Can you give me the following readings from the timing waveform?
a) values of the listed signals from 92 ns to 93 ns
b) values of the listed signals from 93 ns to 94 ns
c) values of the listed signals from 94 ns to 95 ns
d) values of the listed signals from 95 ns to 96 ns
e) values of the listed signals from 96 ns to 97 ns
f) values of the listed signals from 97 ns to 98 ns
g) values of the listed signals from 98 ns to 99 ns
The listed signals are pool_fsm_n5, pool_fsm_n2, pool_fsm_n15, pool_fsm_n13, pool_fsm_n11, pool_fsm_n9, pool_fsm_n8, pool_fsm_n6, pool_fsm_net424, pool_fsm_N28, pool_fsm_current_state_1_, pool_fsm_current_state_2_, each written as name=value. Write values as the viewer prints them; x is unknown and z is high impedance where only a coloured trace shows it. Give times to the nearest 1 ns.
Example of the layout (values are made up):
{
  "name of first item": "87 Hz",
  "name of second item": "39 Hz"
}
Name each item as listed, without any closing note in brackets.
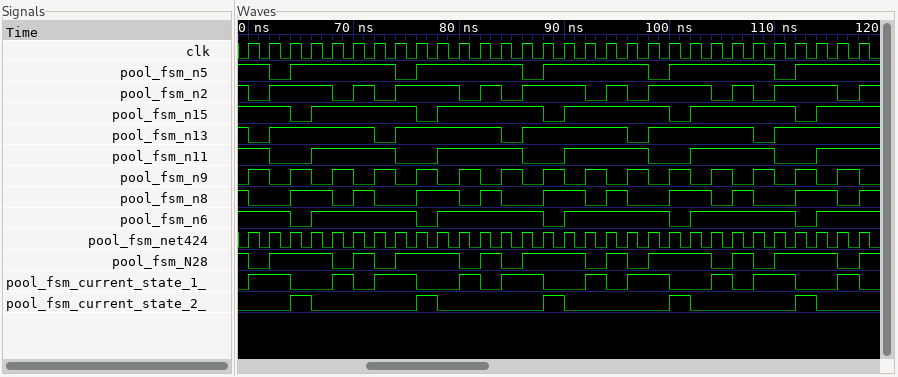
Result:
{
  "values of the listed signals from 92 ns to 93 ns": "pool_fsm_n5=1, pool_fsm_n2=0, pool_fsm_n15=1, pool_fsm_n13=1, pool_fsm_n11=1, pool_fsm_n9=1, pool_fsm_n8=0, pool_fsm_n6=1, pool_fsm_net424=1, pool_fsm_N28=0, pool_fsm_current_state_1_=1, pool_fsm_current_state_2_=0",
  "values of the listed signals from 93 ns to 94 ns": "pool_fsm_n5=1, pool_fsm_n2=0, pool_fsm_n15=1, pool_fsm_n13=1, pool_fsm_n11=1, pool_fsm_n9=1, pool_fsm_n8=0, pool_fsm_n6=1, pool_fsm_net424=0, pool_fsm_N28=0, pool_fsm_current_state_1_=1, pool_fsm_current_state_2_=0",
  "values of the listed signals from 94 ns to 95 ns": "pool_fsm_n5=1, pool_fsm_n2=1, pool_fsm_n15=1, pool_fsm_n13=1, pool_fsm_n11=1, pool_fsm_n9=0, pool_fsm_n8=1, pool_fsm_n6=1, pool_fsm_net424=1, pool_fsm_N28=1, pool_fsm_current_state_1_=0, pool_fsm_current_state_2_=0",
  "values of the listed signals from 95 ns to 96 ns": "pool_fsm_n5=1, pool_fsm_n2=1, pool_fsm_n15=1, pool_fsm_n13=1, pool_fsm_n11=1, pool_fsm_n9=0, pool_fsm_n8=1, pool_fsm_n6=1, pool_fsm_net424=0, pool_fsm_N28=1, pool_fsm_current_state_1_=0, pool_fsm_current_state_2_=0",
  "values of the listed signals from 96 ns to 97 ns": "pool_fsm_n5=1, pool_fsm_n2=0, pool_fsm_n15=1, pool_fsm_n13=0, pool_fsm_n11=1, pool_fsm_n9=1, pool_fsm_n8=0, pool_fsm_n6=1, pool_fsm_net424=1, pool_fsm_N28=0, pool_fsm_current_state_1_=1, pool_fsm_current_state_2_=0",
  "values of the listed signals from 97 ns to 98 ns": "pool_fsm_n5=1, pool_fsm_n2=0, pool_fsm_n15=1, pool_fsm_n13=0, pool_fsm_n11=1, pool_fsm_n9=1, pool_fsm_n8=0, pool_fsm_n6=1, pool_fsm_net424=0, pool_fsm_N28=0, pool_fsm_current_state_1_=1, pool_fsm_current_state_2_=0",
  "values of the listed signals from 98 ns to 99 ns": "pool_fsm_n5=0, pool_fsm_n2=1, pool_fsm_n15=1, pool_fsm_n13=1, pool_fsm_n11=0, pool_fsm_n9=0, pool_fsm_n8=0, pool_fsm_n6=1, pool_fsm_net424=1, pool_fsm_N28=1, pool_fsm_current_state_1_=1, pool_fsm_current_state_2_=0"
}
